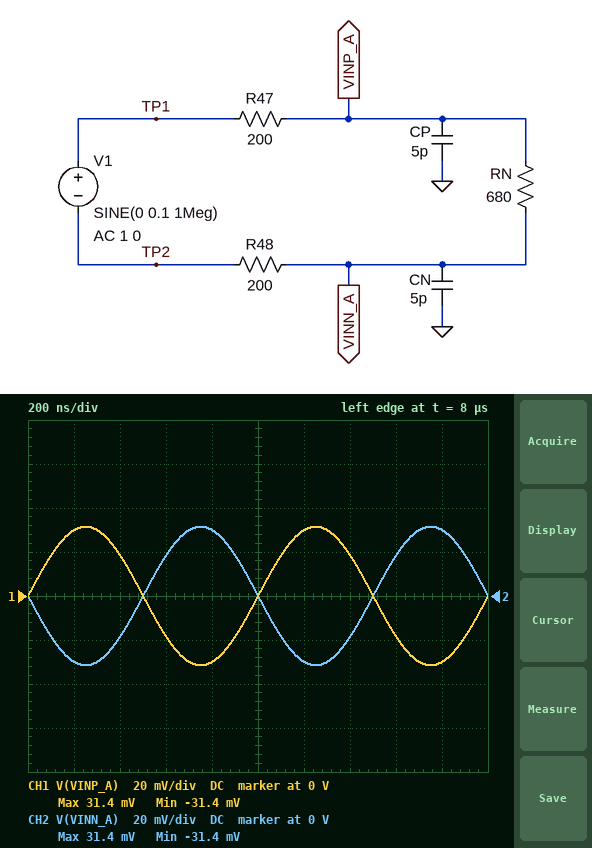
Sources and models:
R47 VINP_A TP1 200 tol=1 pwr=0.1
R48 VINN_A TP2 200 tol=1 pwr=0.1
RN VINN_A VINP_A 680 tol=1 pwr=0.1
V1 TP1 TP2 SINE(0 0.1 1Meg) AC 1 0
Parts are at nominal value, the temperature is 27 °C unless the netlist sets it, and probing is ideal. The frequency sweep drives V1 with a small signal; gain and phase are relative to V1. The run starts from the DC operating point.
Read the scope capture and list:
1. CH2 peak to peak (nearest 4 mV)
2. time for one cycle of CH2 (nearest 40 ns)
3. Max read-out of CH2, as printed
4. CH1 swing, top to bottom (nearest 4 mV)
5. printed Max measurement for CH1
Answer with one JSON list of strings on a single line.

["64 mV", "1.00 µs", "31.4 mV", "64 mV", "31.4 mV"]
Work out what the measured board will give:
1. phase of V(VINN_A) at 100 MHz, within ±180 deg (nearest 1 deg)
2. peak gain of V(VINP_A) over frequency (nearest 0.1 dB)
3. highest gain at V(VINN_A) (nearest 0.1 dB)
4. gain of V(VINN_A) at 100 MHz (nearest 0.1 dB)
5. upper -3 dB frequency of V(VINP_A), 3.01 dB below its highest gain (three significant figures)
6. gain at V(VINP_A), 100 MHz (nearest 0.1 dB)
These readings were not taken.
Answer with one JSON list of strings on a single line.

["158 deg", "-10.0 dB", "-10.0 dB", "-10.7 dB", "253 MHz", "-10.7 dB"]
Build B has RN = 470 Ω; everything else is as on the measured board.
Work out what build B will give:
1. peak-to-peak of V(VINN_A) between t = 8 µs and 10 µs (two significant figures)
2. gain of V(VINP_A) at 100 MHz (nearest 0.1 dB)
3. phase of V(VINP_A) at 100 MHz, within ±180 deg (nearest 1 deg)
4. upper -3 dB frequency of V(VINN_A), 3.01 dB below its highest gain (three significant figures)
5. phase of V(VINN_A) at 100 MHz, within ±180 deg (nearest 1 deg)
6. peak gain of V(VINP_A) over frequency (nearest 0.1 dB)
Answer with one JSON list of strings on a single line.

["54 mV", "-11.8 dB", "-19 deg", "295 MHz", "161 deg", "-11.4 dB"]
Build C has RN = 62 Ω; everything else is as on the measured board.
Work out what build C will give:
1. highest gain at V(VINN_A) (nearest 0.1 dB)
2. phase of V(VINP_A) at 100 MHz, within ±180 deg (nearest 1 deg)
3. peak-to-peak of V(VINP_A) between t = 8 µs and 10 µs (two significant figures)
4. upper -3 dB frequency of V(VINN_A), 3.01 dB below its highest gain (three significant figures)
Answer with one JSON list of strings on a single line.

["-23.5 dB", "-5 deg", "13 mV", "1.19 GHz"]
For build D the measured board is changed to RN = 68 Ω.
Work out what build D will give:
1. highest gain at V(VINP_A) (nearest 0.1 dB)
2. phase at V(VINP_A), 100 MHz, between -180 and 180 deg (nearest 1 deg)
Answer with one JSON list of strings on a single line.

["-22.8 dB", "-5 deg"]
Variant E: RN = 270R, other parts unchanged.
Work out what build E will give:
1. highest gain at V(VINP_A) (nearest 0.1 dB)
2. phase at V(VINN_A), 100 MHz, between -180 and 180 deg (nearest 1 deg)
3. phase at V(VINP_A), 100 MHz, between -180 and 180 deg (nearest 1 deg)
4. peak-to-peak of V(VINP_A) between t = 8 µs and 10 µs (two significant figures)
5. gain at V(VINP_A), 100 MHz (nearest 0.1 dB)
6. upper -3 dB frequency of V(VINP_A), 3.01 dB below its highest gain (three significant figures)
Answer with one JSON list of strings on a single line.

["-13.9 dB", "166 deg", "-14 deg", "40 mV", "-14.2 dB", "395 MHz"]
